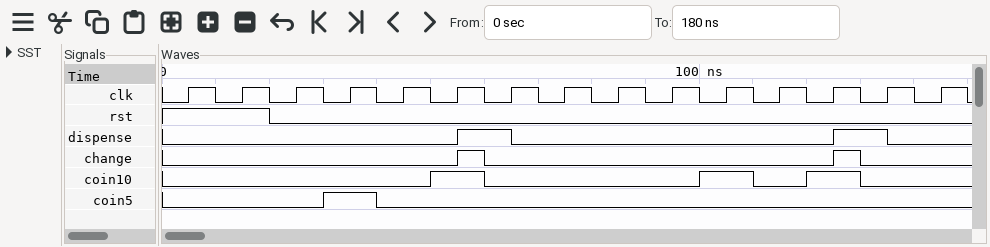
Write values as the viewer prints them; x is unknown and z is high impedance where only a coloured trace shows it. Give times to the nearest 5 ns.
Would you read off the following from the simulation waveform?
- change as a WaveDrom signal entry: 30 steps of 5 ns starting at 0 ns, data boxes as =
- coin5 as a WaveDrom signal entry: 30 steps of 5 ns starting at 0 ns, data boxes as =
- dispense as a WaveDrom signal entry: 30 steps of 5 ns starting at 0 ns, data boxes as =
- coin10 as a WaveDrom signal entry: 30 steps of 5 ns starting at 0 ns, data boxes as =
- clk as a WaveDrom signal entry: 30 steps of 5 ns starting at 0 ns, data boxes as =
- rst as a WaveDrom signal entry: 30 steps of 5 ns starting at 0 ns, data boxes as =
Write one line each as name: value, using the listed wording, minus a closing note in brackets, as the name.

change as a WaveDrom signal entry: 30 steps of 5 ns starting at 0 ns, data boxes as =: {name: 'change', wave: '0..........10............10...'}
coin5 as a WaveDrom signal entry: 30 steps of 5 ns starting at 0 ns, data boxes as =: {name: 'coin5', wave: '0.....1.0.....................'}
dispense as a WaveDrom signal entry: 30 steps of 5 ns starting at 0 ns, data boxes as =: {name: 'dispense', wave: '0..........1.0...........1.0..'}
coin10 as a WaveDrom signal entry: 30 steps of 5 ns starting at 0 ns, data boxes as =: {name: 'coin10', wave: '0.........1.0.......1.0.1.0...'}
clk as a WaveDrom signal entry: 30 steps of 5 ns starting at 0 ns, data boxes as =: {name: 'clk', wave: '010101010101010101010101010101'}
rst as a WaveDrom signal entry: 30 steps of 5 ns starting at 0 ns, data boxes as =: {name: 'rst', wave: '1...0.........................'}
